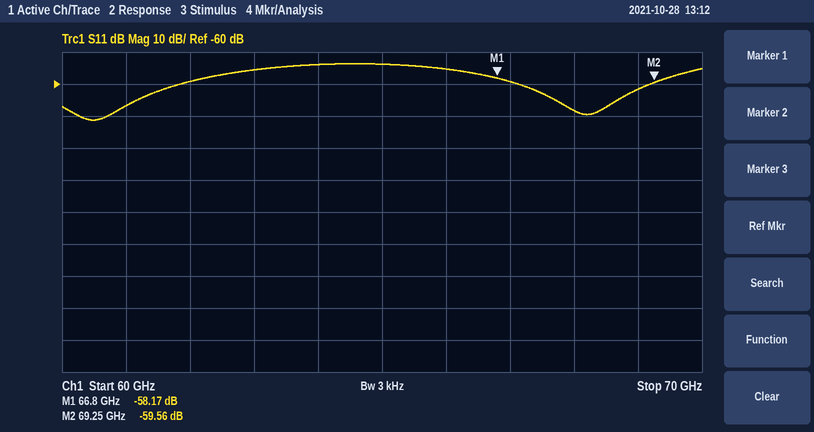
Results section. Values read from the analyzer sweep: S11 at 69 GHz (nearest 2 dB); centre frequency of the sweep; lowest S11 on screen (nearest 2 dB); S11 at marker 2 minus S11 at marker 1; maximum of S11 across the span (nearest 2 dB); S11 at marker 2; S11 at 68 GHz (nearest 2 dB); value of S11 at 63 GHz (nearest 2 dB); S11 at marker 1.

-62 dB
65 GHz
-72 dB
-1.39 dB
-54 dB
-59.56 dB
-68 dB
-56 dB
-58.17 dB
